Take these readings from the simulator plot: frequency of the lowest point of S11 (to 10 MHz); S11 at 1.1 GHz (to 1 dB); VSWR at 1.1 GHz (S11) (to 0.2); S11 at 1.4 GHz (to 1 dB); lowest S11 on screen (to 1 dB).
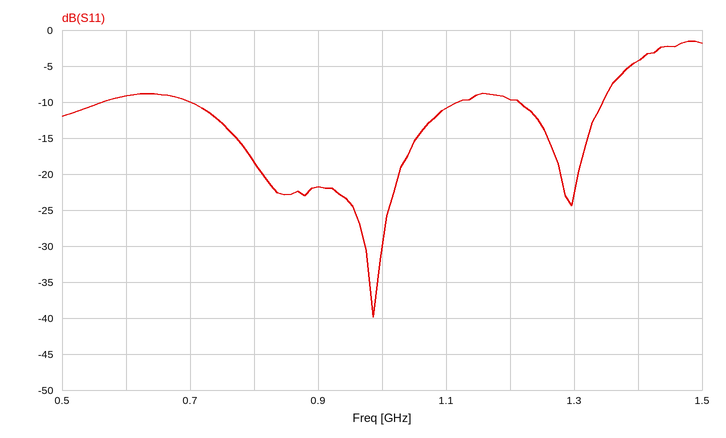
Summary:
990 MHz
-11 dB
1.8
-4 dB
-40 dB
